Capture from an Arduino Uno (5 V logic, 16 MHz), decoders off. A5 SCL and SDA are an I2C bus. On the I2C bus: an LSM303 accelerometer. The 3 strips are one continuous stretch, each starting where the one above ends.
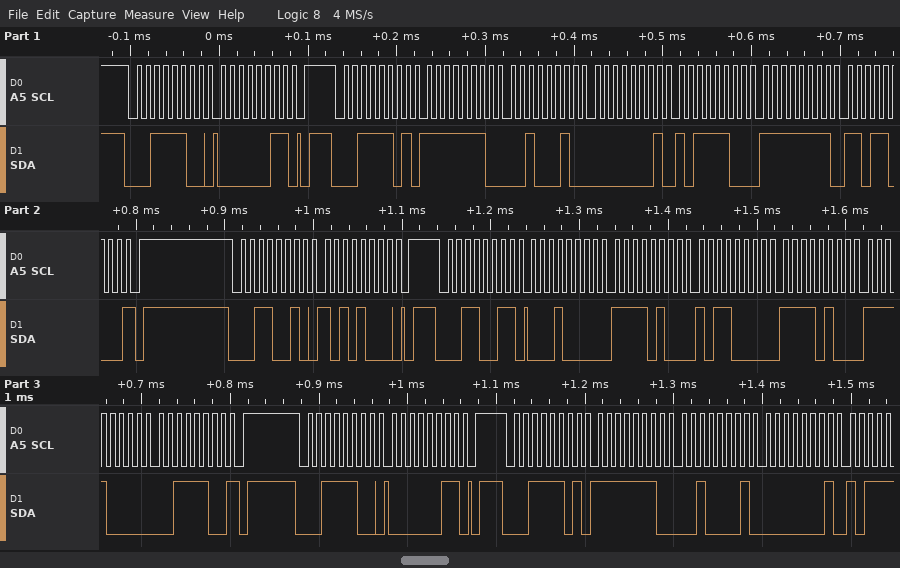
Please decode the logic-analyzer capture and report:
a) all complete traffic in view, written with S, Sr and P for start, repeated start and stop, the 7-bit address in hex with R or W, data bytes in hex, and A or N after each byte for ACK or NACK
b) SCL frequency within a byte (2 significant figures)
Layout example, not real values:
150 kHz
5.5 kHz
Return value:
S 1EW A 03 A P S 1ER A FE A 22 A 01 A BC A FF A D8 N P S 19W A A8 A P S 19R A 10 A F4 A B0 A F4 A F0 A 3C N P S 1EW A 03 A P S 1ER A FE A 21 A 01 A
100 kHz
